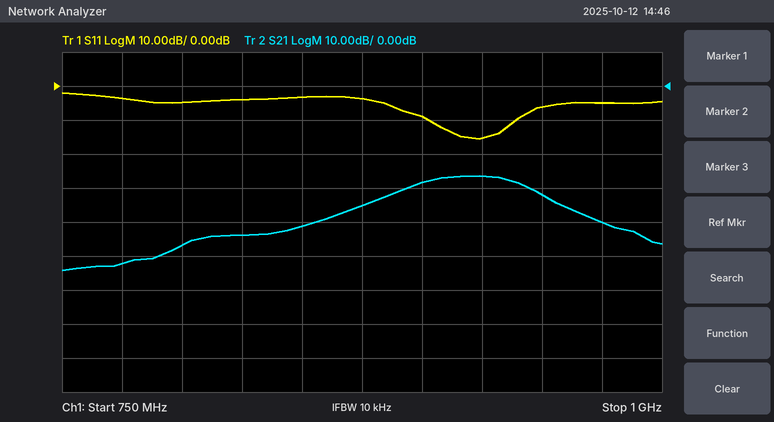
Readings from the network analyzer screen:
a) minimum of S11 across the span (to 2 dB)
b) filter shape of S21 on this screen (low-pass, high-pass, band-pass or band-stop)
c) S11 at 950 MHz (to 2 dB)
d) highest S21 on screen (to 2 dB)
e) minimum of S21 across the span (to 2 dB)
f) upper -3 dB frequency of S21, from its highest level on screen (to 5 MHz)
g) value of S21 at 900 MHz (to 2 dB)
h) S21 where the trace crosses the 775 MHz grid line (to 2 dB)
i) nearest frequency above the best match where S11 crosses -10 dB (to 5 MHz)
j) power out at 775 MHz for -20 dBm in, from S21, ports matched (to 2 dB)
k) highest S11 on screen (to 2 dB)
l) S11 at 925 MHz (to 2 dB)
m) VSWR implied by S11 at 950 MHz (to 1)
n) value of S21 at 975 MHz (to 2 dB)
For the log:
-16 dB
band-pass
-6 dB
-26 dB
-54 dB
945 MHz
-28 dB
-52 dB
940 MHz
-72 dBm
-2 dB
-16 dB
3
-40 dB
